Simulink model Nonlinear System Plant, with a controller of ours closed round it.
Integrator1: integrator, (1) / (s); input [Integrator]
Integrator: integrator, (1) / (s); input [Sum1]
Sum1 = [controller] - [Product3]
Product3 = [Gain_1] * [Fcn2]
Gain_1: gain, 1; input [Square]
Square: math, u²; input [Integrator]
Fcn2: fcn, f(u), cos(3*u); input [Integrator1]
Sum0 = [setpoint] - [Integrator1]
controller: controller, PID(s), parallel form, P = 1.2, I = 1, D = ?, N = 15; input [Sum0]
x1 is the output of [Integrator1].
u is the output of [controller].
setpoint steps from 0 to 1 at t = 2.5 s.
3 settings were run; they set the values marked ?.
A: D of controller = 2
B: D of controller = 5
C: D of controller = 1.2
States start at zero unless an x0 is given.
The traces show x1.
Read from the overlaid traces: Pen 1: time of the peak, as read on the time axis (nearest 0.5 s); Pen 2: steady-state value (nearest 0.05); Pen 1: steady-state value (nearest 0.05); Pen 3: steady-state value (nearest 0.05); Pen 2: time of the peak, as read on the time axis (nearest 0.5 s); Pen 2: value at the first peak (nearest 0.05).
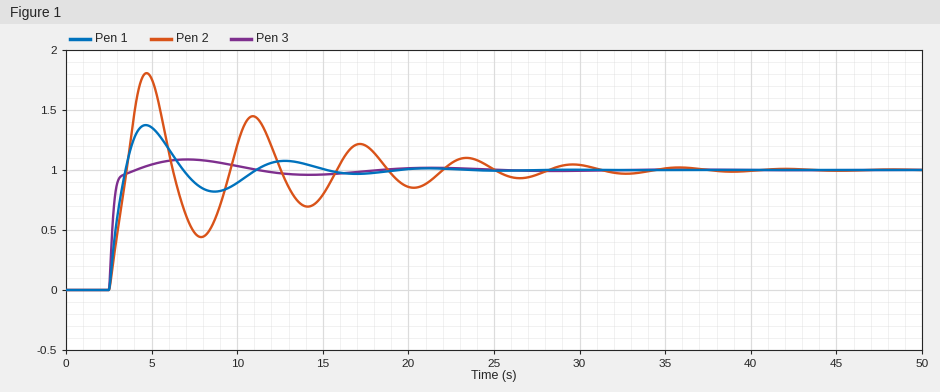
4.5 s
1.00
1.00
1.00
4.5 s
1.80
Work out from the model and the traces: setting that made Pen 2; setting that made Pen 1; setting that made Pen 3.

C
A
B
